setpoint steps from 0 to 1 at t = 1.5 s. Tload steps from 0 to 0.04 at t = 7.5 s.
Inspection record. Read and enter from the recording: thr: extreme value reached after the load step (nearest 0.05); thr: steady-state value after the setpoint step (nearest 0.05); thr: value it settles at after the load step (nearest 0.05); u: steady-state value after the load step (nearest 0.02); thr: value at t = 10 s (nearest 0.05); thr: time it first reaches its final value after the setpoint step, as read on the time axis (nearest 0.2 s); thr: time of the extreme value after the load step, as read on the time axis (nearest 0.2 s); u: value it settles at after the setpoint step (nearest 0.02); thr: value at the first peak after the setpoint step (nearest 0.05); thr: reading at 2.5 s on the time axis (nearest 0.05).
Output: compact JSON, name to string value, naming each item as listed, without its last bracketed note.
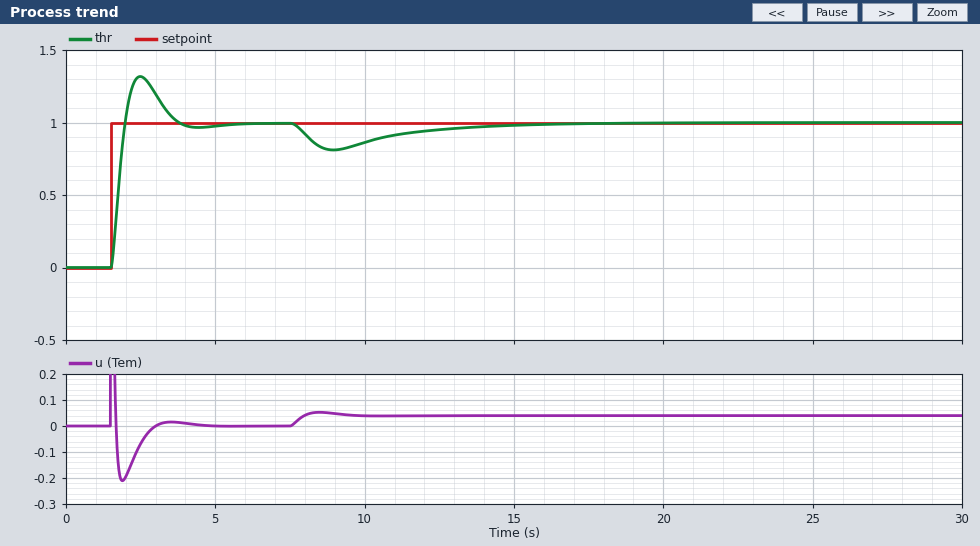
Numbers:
{"thr: extreme value reached after the load step": "0.80", "thr: steady-state value after the setpoint step": "1.00", "thr: value it settles at after the load step": "1.00", "u: steady-state value after the load step": "0.04", "thr: value at t = 10 s": "0.85", "thr: time it first reaches its final value after the setpoint step, as read on the time axis": "2.0 s", "thr: time of the extreme value after the load step, as read on the time axis": "9.0 s", "u: value it settles at after the setpoint step": "0.00", "thr: value at the first peak after the setpoint step": "1.30", "thr: reading at 2.5 s on the time axis": "1.30"}
